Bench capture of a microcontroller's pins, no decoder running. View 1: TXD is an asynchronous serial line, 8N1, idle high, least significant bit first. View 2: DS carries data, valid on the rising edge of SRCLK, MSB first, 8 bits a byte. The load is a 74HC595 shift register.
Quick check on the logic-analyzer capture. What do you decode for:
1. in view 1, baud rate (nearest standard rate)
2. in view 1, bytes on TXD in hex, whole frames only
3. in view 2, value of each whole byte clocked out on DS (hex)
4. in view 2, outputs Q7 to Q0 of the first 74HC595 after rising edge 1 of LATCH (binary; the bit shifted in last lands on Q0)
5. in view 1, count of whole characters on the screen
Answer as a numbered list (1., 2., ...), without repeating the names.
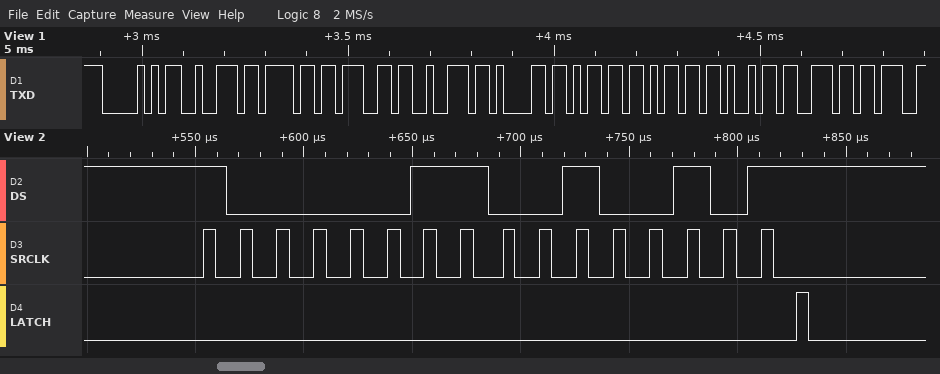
1. 57600 baud
2. 0x50 0x72 0x6F 0x67 0x72 0x61 0x6D 0x6D 0x69 0x6E
3. 83 25
4. 00100101
5. 10
